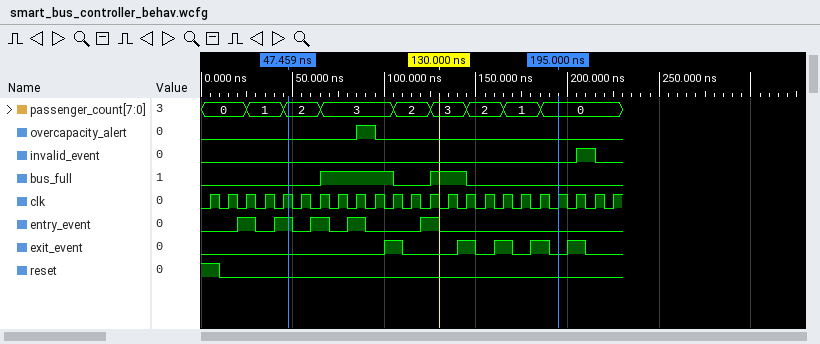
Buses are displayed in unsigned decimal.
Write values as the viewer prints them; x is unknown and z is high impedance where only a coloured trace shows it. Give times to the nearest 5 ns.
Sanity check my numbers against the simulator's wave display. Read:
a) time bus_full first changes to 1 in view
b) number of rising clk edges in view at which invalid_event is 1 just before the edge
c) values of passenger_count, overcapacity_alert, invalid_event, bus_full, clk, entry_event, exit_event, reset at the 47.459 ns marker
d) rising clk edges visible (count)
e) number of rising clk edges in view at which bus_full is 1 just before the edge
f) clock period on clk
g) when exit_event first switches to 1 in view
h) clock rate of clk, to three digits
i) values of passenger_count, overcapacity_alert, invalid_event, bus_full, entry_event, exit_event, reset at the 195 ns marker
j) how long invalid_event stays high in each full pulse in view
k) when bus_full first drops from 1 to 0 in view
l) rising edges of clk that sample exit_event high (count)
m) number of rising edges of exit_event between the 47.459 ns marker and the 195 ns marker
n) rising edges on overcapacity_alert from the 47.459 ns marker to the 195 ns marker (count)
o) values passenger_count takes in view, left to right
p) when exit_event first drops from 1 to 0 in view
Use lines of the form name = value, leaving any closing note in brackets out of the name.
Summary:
time bus_full first changes to 1 in view = 65 ns
number of rising clk edges in view at which invalid_event is 1 just before the edge = 1
values of passenger_count, overcapacity_alert, invalid_event, bus_full, clk, entry_event, exit_event, reset at the 47.459 ns marker = passenger_count=2, overcapacity_alert=0, invalid_event=0, bus_full=0, clk=1, entry_event=1, exit_event=0, reset=0
rising clk edges visible = 23
number of rising clk edges in view at which bus_full is 1 just before the edge = 6
clock period on clk = 10 ns
when exit_event first switches to 1 in view = 100 ns
clock rate of clk, to three digits = 100 MHz
values of passenger_count, overcapacity_alert, invalid_event, bus_full, entry_event, exit_event, reset at the 195 ns marker = passenger_count=0, overcapacity_alert=0, invalid_event=0, bus_full=0, entry_event=0, exit_event=0, reset=0
how long invalid_event stays high in each full pulse in view = 10 ns
when bus_full first drops from 1 to 0 in view = 105 ns
rising edges of clk that sample exit_event high = 5
number of rising edges of exit_event between the 47.459 ns marker and the 195 ns marker = 4
rising edges on overcapacity_alert from the 47.459 ns marker to the 195 ns marker = 1
values passenger_count takes in view, left to right = 0, 1, 2, 3, 2, 3, 2, 1, 0
when exit_event first drops from 1 to 0 in view = 110 ns
